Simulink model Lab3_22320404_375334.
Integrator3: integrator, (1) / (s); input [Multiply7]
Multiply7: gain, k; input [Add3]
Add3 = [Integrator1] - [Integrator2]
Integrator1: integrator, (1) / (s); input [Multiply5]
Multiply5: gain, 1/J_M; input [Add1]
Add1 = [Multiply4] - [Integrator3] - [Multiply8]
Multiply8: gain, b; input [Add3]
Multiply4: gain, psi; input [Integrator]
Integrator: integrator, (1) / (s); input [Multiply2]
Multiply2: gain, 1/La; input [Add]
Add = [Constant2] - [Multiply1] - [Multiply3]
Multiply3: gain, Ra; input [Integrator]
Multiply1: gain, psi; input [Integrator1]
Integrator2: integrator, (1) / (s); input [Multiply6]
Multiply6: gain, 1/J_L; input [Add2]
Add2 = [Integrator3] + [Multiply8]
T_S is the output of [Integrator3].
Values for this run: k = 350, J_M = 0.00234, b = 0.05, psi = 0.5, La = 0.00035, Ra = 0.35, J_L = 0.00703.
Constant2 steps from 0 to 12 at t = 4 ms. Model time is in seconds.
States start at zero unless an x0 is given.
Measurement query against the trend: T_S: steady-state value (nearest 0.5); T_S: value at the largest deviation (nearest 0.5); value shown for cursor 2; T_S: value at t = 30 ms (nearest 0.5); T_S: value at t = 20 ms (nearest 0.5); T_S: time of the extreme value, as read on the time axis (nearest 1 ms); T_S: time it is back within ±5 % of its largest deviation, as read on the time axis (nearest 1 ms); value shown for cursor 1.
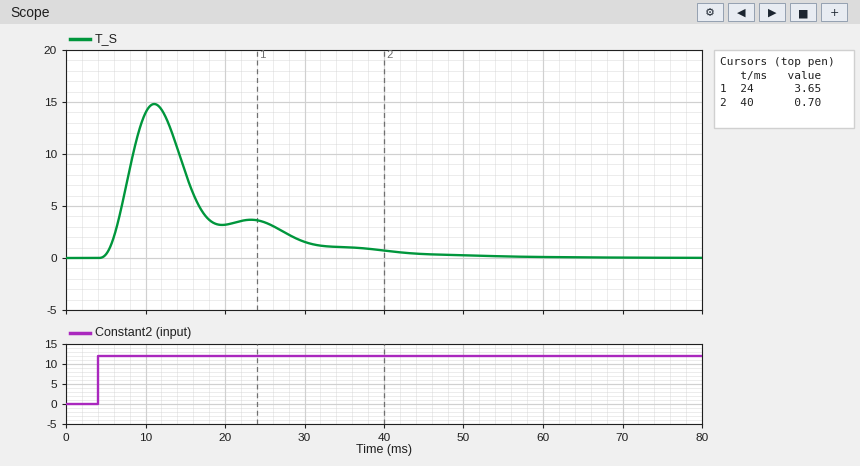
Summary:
0.0
15.0
0.70
1.5
3.0
11 ms
40 ms
3.65
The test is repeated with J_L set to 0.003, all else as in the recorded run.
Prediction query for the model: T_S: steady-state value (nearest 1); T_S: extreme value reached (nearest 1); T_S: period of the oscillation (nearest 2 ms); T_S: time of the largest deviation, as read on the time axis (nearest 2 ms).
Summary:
0
11
12 ms
10 ms
